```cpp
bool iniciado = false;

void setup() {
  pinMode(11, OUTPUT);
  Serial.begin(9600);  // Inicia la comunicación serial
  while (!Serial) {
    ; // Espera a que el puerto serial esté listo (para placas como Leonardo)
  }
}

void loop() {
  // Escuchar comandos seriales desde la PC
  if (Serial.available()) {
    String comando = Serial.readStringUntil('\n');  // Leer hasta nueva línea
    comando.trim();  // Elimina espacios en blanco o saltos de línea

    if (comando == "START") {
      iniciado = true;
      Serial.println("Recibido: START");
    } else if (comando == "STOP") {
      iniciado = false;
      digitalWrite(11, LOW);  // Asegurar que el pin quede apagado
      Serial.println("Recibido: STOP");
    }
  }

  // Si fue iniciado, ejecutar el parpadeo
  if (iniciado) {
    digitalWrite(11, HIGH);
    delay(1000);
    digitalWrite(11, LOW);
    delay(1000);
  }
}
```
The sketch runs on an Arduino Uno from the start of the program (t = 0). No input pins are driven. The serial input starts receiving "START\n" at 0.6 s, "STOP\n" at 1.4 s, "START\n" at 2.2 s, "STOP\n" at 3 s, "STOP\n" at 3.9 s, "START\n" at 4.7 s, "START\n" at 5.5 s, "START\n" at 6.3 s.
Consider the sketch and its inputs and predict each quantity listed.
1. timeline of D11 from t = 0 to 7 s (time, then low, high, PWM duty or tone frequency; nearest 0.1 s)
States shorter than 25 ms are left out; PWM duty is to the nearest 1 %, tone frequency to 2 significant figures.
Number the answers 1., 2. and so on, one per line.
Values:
1. 0 s low; 0.6 s high; 1.6 s low; 2.6 s high; 3.6 s low; 4.7 s high; 5.7 s low; 6.7 s high
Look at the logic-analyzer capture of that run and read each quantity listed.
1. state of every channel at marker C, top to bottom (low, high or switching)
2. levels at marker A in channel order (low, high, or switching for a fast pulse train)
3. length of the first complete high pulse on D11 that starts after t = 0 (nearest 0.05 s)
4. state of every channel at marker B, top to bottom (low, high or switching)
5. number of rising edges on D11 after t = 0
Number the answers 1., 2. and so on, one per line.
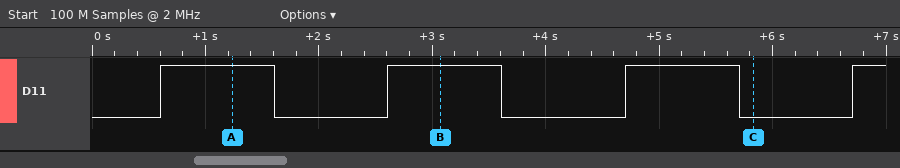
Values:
1. D11 low
2. D11 high
3. 1.00 s
4. D11 high
5. 4
